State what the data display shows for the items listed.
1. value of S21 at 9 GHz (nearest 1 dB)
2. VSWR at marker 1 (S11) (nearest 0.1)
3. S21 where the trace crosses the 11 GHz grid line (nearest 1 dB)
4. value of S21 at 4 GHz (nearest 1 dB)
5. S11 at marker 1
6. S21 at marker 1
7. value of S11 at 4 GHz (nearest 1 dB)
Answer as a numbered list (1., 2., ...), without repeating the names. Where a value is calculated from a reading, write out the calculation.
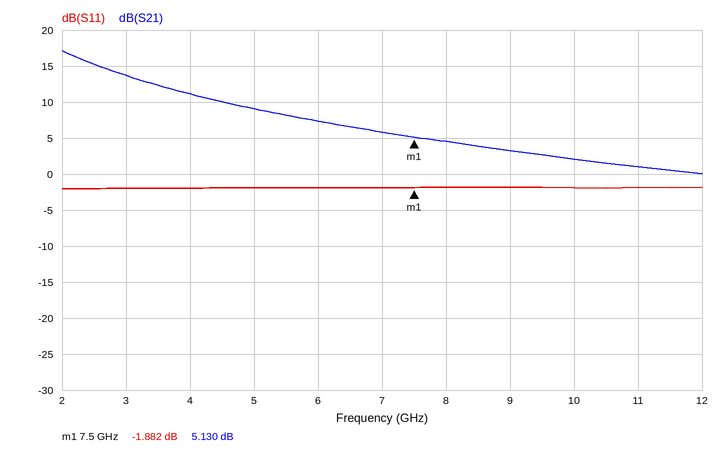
1. 3 dB
2. (1 + 0.8052)/(1 − 0.8052) ≈ 9.3
3. 1 dB
4. 11 dB
5. -1.882 dB
6. 5.130 dB
7. -2 dB
